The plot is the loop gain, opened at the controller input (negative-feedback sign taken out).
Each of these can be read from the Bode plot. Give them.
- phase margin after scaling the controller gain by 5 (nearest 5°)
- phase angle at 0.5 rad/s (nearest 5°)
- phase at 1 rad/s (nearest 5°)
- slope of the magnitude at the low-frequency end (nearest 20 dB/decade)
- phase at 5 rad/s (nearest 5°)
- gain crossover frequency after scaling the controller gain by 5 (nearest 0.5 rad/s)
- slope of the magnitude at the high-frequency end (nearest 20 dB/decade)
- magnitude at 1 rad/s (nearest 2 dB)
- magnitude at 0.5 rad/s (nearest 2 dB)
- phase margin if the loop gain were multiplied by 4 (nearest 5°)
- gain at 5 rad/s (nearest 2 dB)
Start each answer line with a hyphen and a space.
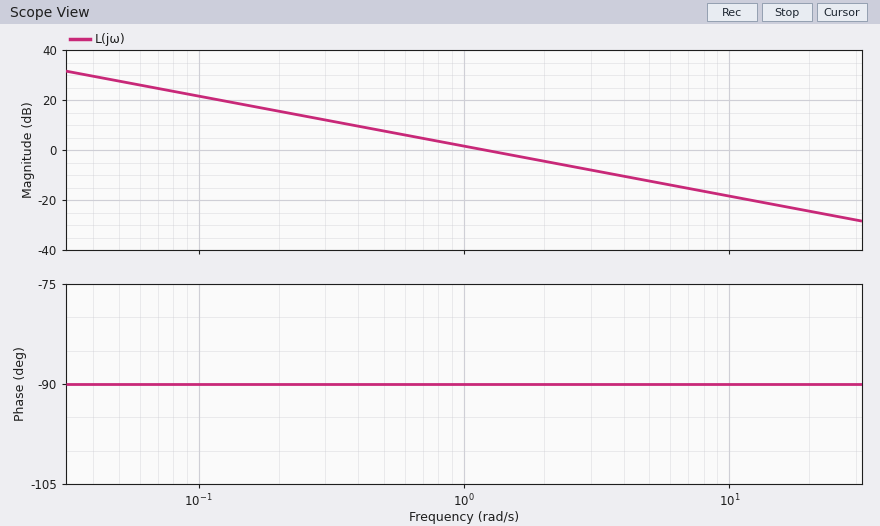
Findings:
- 90°
- -90°
- -90°
- -20 dB/decade
- -90°
- 6.0 rad/s
- -20 dB/decade
- 2 dB
- 8 dB
- 90°
- -12 dB
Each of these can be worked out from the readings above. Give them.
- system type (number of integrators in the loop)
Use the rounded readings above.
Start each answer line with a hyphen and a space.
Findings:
- 1
